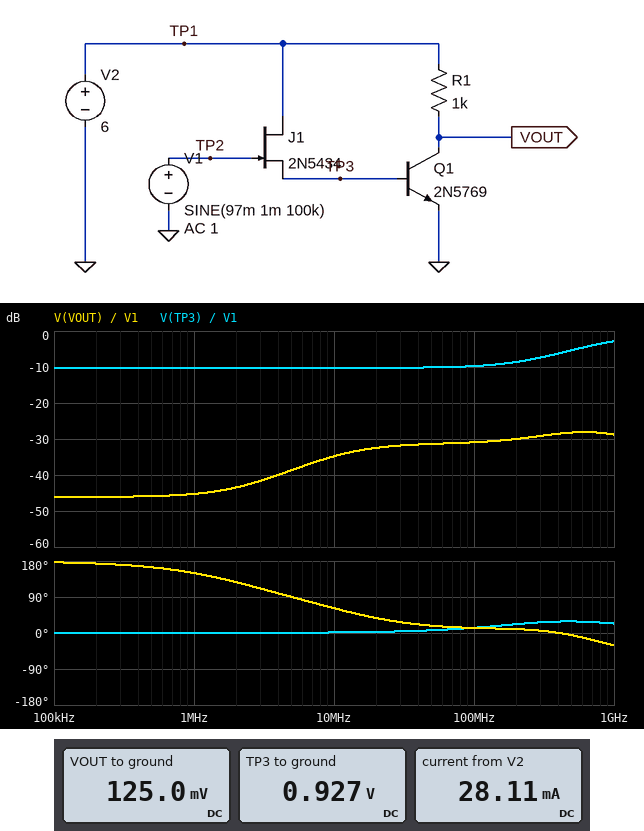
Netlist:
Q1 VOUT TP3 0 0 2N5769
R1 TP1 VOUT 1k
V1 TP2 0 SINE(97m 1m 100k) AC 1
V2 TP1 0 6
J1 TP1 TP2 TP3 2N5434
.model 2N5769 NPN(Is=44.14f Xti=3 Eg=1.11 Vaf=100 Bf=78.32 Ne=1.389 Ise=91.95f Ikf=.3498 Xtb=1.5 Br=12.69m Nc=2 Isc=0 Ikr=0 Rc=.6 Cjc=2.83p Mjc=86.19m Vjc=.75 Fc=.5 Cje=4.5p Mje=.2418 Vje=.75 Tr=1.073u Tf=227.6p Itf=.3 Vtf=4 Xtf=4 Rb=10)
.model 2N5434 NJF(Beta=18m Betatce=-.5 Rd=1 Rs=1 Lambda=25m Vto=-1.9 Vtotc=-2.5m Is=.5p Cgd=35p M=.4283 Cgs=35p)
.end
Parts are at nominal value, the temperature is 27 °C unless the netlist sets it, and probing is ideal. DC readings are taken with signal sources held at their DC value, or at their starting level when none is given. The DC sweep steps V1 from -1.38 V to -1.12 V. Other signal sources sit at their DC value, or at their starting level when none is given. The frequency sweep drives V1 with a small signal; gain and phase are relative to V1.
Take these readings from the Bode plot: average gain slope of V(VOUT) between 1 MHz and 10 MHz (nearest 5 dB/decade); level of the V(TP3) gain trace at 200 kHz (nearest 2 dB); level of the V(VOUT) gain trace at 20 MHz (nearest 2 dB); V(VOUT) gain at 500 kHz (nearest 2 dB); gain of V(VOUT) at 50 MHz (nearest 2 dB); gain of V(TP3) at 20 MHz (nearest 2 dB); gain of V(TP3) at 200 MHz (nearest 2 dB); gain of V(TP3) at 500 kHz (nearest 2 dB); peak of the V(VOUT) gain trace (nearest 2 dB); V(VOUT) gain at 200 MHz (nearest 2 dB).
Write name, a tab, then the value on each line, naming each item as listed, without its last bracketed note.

average gain slope of V(VOUT) between 1 MHz and 10 MHz	10 dB/decade
level of the V(TP3) gain trace at 200 kHz	-10 dB
level of the V(VOUT) gain trace at 20 MHz	-32 dB
V(VOUT) gain at 500 kHz	-46 dB
gain of V(VOUT) at 50 MHz	-32 dB
gain of V(TP3) at 20 MHz	-10 dB
gain of V(TP3) at 200 MHz	-8 dB
gain of V(TP3) at 500 kHz	-10 dB
peak of the V(VOUT) gain trace	-28 dB
V(VOUT) gain at 200 MHz	-30 dB
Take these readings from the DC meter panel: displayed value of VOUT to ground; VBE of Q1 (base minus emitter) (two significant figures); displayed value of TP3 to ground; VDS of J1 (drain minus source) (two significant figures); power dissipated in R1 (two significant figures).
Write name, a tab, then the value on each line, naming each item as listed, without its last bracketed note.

displayed value of VOUT to ground	125.0 mV
VBE of Q1 (base minus emitter)	930 mV
displayed value of TP3 to ground	0.927 V
VDS of J1 (drain minus source)	5.1 V
power dissipated in R1	35 mW
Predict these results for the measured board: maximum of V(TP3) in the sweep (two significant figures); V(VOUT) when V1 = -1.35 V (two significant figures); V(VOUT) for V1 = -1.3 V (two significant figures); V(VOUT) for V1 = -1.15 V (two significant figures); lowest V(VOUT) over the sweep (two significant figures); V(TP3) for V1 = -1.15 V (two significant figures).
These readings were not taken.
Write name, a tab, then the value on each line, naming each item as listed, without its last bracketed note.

maximum of V(TP3) in the sweep	670 mV
V(VOUT) when V1 = -1.35 V	5.9 V
V(VOUT) for V1 = -1.3 V	5.7 V
V(VOUT) for V1 = -1.15 V	230 mV
lowest V(VOUT) over the sweep	210 mV
V(TP3) for V1 = -1.15 V	660 mV
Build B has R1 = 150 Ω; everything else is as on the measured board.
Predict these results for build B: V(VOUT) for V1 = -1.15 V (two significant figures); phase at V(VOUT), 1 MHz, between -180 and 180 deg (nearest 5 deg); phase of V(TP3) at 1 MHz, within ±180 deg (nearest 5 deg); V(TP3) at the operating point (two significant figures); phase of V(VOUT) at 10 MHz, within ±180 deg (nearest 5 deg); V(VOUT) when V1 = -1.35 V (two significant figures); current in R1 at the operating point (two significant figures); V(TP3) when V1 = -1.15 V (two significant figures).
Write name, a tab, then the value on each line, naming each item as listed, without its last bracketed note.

V(VOUT) for V1 = -1.15 V	4.7 V
phase at V(VOUT), 1 MHz, between -180 and 180 deg	170 deg
phase of V(TP3) at 1 MHz, within ±180 deg	0 deg
V(TP3) at the operating point	940 mV
phase of V(VOUT) at 10 MHz, within ±180 deg	110 deg
V(VOUT) when V1 = -1.35 V	6.0 V
current in R1 at the operating point	39 mA
V(TP3) when V1 = -1.15 V	670 mV
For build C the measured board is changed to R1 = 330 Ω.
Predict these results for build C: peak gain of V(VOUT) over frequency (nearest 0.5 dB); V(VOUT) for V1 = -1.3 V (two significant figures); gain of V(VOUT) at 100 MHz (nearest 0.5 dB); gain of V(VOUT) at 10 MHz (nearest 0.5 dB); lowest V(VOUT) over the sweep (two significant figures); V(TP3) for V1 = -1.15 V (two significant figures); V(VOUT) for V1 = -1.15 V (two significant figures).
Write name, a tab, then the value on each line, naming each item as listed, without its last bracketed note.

peak gain of V(VOUT) over frequency	-31.0 dB
V(VOUT) for V1 = -1.3 V	5.9 V
gain of V(VOUT) at 100 MHz	-33.5 dB
gain of V(VOUT) at 10 MHz	-35.5 dB
lowest V(VOUT) over the sweep	1.8 V
V(TP3) for V1 = -1.15 V	670 mV
V(VOUT) for V1 = -1.15 V	3.2 V
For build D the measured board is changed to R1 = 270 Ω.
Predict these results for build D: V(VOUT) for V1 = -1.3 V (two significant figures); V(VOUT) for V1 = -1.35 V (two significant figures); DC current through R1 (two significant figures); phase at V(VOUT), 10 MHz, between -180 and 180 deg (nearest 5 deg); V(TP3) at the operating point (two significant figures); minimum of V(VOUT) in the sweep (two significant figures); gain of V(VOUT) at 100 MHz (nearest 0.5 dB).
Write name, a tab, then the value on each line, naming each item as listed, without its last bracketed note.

V(VOUT) for V1 = -1.3 V	5.9 V
V(VOUT) for V1 = -1.35 V	6.0 V
DC current through R1	22 mA
phase at V(VOUT), 10 MHz, between -180 and 180 deg	95 deg
V(TP3) at the operating point	940 mV
minimum of V(VOUT) in the sweep	2.5 V
gain of V(VOUT) at 100 MHz	-34.5 dB
